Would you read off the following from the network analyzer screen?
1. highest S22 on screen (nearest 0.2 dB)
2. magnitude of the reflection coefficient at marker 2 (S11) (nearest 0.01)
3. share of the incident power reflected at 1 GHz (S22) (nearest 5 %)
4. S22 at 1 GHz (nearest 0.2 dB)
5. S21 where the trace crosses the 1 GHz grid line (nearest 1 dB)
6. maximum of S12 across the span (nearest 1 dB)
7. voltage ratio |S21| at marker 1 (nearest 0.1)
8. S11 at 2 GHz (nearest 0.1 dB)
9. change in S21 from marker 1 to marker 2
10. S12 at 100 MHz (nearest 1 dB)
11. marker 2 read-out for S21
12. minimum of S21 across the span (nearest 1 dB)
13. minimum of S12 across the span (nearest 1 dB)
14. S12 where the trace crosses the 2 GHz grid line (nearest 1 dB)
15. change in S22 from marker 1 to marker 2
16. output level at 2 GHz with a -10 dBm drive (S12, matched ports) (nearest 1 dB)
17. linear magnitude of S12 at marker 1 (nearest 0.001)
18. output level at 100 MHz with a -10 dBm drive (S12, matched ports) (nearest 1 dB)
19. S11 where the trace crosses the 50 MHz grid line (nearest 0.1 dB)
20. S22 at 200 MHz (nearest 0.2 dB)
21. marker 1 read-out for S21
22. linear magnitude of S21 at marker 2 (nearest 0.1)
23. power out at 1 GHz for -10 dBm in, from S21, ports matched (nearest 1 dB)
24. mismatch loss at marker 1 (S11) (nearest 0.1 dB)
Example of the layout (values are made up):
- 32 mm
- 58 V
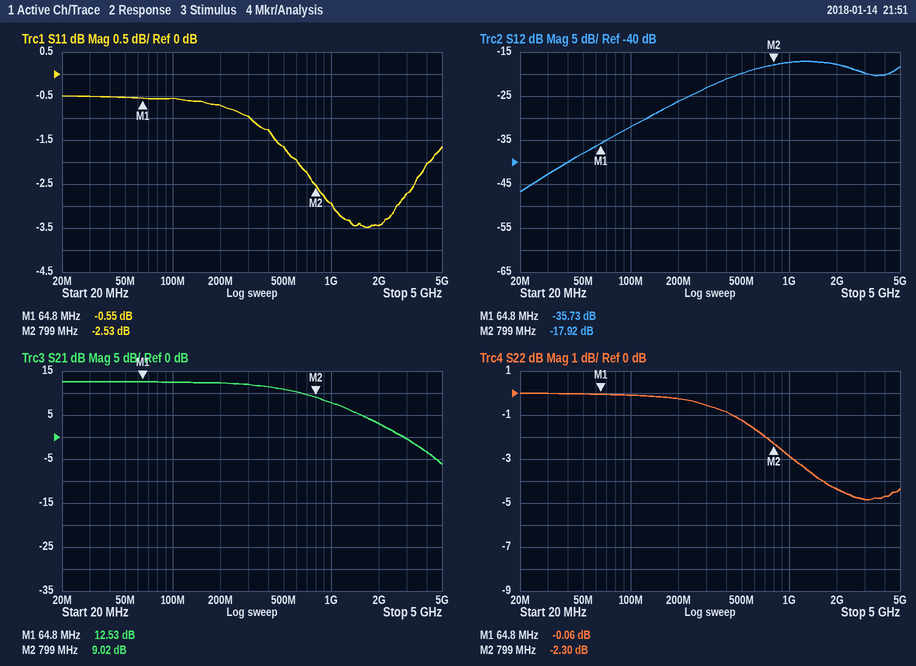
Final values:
- 0.0 dB
- 0.75
- 50 %
- -2.8 dB
- 8 dB
- -17 dB
- 4.2
- -3.4 dB
- -3.51 dB
- -32 dB
- 9.02 dB
- -6 dB
- -47 dB
- -18 dB
- -2.24 dB
- -28 dBm
- 0.016
- -42 dBm
- -0.5 dB
- -0.2 dB
- 12.53 dB
- 2.8
- -2 dBm
- 9.2 dB
